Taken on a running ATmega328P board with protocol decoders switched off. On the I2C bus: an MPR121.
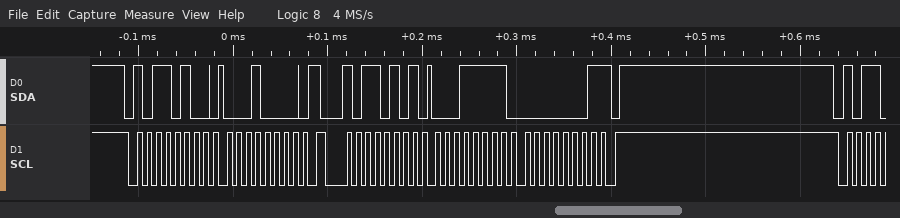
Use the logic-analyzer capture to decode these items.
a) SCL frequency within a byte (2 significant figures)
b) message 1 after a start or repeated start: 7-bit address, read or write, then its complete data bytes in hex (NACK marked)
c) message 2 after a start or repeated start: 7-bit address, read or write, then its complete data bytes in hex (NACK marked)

100 kHz
0x5A write: 10
0x5A read: 1F 01 NACK
